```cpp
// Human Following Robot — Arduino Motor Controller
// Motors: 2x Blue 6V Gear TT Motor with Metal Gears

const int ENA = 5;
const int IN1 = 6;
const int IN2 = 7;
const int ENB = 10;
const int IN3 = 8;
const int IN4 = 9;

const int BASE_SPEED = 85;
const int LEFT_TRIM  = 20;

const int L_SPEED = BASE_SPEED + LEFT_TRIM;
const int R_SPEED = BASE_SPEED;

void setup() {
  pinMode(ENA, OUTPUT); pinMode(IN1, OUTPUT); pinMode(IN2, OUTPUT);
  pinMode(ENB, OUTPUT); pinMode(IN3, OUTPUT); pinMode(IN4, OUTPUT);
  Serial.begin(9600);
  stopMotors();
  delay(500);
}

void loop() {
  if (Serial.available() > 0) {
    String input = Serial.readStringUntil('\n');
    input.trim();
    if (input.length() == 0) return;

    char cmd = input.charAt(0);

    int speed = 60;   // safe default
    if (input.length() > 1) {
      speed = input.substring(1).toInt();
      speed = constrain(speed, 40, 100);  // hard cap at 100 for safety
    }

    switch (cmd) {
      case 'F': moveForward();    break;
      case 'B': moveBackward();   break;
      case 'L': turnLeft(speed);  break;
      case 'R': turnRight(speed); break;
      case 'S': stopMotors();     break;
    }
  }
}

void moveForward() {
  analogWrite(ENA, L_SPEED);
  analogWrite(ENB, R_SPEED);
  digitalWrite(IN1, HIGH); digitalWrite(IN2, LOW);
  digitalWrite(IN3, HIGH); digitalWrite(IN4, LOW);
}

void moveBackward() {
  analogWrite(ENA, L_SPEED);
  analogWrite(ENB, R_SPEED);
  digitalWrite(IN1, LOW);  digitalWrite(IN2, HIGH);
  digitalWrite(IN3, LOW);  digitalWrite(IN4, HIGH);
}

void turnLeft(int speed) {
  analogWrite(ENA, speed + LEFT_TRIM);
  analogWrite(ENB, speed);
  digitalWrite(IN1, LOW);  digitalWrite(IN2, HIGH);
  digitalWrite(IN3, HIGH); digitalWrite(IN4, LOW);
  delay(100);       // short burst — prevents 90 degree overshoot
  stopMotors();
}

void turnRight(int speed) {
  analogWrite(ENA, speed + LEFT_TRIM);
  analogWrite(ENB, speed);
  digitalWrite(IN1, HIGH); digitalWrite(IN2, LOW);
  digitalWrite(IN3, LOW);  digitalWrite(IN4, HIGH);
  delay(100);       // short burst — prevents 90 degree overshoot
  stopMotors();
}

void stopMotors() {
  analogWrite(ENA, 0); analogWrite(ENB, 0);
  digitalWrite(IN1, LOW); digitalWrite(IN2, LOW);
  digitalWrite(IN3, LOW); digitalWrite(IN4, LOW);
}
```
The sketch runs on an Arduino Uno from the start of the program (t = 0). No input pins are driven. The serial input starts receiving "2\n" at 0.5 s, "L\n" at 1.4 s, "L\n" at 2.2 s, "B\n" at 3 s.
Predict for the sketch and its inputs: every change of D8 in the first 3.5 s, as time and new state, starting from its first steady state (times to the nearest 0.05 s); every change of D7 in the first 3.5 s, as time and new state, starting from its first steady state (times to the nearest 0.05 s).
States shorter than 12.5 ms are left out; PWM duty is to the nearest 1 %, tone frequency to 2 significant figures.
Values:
0 s low; 1.4 s high; 1.5 s low; 2.2 s high; 2.3 s low
0 s low; 1.4 s high; 1.5 s low; 2.2 s high; 2.3 s low; 3 s high
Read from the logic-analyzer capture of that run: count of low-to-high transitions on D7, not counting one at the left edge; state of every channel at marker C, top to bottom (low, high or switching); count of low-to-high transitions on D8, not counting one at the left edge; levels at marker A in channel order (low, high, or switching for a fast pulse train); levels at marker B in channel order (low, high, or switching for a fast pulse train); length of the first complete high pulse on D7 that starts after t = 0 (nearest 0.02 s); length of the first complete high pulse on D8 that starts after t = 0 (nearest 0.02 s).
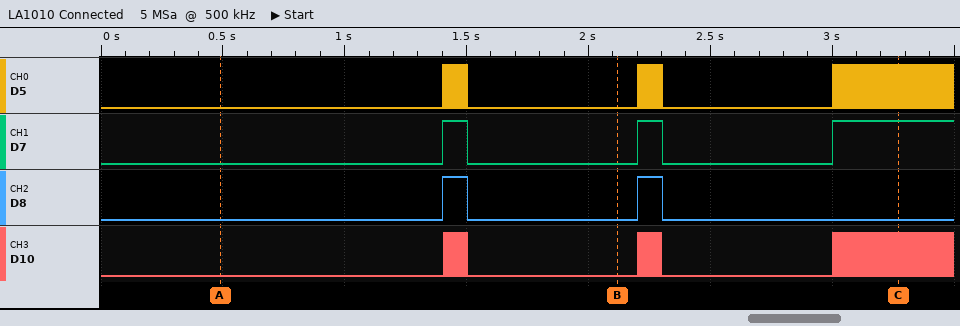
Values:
3
D5 switching, D7 high, D8 low, D10 switching
2
D5 low, D7 low, D8 low, D10 low
D5 low, D7 low, D8 low, D10 low
0.10 s
0.10 s
